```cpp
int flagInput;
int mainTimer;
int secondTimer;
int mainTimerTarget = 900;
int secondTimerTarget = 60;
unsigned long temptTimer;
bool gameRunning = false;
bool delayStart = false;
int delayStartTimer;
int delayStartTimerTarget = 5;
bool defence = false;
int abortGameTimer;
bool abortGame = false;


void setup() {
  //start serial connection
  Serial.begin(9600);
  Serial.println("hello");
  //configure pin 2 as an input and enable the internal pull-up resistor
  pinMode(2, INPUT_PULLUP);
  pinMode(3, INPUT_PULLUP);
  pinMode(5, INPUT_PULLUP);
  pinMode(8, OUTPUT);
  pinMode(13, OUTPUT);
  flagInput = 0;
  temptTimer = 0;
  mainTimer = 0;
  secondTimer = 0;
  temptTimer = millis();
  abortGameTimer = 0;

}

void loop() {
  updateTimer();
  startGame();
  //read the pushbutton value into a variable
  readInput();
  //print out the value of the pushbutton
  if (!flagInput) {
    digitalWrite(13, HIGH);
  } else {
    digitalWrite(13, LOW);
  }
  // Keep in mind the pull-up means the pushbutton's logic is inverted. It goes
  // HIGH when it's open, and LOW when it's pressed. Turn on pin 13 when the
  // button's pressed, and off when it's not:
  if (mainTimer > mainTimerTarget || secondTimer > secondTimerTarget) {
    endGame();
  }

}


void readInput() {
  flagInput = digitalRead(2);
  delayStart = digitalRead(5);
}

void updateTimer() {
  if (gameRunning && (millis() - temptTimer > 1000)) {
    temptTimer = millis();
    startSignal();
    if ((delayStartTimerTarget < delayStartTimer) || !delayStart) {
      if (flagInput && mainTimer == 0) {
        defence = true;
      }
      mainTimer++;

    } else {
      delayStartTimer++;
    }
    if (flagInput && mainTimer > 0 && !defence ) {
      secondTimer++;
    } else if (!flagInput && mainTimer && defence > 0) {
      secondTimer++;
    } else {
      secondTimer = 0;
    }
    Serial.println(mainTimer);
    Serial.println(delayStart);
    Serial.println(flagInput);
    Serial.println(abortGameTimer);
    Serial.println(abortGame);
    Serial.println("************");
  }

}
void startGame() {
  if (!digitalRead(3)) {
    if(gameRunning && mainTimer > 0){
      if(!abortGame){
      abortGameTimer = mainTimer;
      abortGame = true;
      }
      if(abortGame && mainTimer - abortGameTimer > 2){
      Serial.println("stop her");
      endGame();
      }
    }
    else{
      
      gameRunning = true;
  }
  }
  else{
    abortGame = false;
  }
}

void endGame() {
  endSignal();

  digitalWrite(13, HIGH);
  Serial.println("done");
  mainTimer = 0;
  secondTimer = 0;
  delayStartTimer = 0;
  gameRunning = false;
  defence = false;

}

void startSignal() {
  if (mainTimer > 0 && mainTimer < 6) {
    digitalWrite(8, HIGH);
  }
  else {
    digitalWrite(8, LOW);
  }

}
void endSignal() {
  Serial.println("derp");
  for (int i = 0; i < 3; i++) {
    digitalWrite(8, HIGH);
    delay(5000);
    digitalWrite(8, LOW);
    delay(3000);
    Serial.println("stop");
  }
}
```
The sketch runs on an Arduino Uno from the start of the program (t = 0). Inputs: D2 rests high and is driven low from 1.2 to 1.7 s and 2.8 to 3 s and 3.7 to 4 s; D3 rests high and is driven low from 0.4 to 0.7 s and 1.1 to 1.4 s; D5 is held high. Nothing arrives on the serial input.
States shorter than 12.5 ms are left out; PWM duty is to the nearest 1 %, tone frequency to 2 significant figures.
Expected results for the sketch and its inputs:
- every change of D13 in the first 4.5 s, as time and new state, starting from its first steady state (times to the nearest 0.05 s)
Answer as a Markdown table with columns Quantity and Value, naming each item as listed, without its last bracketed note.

| Quantity | Value |
|---|---|
| every change of D13 in the first 4.5 s, as time and new state, starting from its first steady state | 0 s low; 1.2 s high; 1.7 s low; 2.8 s high; 3 s low; 3.7 s high; 4 s low |
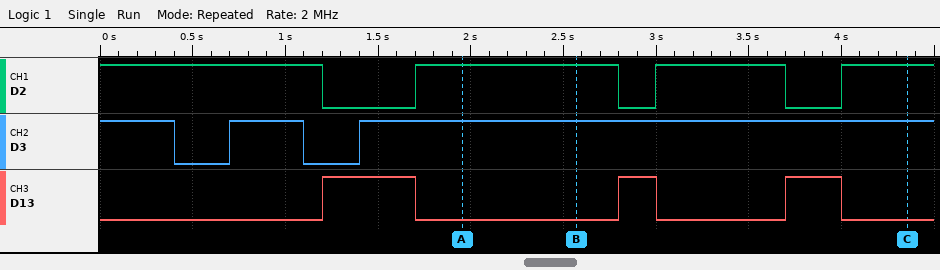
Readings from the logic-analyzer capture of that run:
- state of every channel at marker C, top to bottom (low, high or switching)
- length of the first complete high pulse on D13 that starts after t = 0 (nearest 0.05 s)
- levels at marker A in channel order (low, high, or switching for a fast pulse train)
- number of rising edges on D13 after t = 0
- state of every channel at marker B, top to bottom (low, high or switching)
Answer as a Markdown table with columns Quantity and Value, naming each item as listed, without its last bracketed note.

| Quantity | Value |
|---|---|
| state of every channel at marker C, top to bottom | D2 high, D3 high, D13 low |
| length of the first complete high pulse on D13 that starts after t = 0 | 0.50 s |
| levels at marker A in channel order | D2 high, D3 high, D13 low |
| number of rising edges on D13 after t = 0 | 3 |
| state of every channel at marker B, top to bottom | D2 high, D3 high, D13 low |
